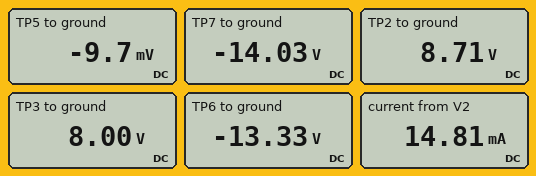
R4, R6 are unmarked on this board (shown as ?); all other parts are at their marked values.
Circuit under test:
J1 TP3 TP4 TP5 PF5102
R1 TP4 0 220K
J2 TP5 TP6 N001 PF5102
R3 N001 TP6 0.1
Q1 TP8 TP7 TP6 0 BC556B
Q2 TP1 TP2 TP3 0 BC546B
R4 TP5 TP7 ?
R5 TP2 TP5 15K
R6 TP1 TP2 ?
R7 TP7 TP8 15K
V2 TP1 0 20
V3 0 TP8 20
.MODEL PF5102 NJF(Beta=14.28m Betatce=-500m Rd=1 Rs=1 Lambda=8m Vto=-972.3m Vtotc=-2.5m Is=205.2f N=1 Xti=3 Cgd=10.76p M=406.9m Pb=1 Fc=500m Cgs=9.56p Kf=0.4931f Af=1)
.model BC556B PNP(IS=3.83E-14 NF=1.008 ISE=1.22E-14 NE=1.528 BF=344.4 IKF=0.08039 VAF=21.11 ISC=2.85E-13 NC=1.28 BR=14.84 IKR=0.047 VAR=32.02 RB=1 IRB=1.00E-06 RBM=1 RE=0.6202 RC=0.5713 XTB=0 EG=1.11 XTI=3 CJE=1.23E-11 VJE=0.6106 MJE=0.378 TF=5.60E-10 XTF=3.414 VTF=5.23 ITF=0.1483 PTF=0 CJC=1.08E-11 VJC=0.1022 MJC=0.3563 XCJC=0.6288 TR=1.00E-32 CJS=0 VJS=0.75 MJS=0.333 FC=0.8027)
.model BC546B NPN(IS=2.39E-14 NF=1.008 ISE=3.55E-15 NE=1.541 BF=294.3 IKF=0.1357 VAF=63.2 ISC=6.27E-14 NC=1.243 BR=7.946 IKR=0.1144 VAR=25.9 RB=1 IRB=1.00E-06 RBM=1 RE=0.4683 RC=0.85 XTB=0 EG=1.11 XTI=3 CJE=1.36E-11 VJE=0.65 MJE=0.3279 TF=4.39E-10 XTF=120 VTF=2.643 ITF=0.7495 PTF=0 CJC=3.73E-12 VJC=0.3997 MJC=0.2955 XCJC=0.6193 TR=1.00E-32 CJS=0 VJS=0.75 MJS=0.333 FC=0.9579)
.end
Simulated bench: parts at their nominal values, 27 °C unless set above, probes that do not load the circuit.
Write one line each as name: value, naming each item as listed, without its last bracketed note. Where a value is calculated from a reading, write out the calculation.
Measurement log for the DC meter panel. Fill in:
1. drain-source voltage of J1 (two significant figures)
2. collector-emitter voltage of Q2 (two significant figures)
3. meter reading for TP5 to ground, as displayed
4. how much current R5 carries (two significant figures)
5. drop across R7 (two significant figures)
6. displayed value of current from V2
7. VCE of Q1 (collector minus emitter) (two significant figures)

drain-source voltage of J1: 8 V - (-9.7 mV) = 8.0 V
collector-emitter voltage of Q2: 20 V - 8 V = 12 V
meter reading for TP5 to ground, as displayed: -9.7 mV
how much current R5 carries: (8.71 V - (-9.7 mV)) / 15 kΩ = 580 µA
drop across R7: -14.03 V - (-20 V) = 6.0 V
displayed value of current from V2: 14.81 mA
VCE of Q1 (collector minus emitter): -20 V - (-13.33 V) = -6.7 V
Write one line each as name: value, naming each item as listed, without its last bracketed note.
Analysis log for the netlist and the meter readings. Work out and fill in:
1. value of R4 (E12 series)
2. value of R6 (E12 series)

value of R4: 39 kΩ
value of R6: 18 kΩ
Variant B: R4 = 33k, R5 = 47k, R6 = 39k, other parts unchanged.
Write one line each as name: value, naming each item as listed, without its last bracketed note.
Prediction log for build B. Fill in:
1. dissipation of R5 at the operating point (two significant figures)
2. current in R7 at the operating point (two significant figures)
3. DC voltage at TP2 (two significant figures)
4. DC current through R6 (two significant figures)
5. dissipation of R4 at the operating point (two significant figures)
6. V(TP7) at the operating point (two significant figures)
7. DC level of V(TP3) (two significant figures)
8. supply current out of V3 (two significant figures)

dissipation of R5 at the operating point: 2.1 mW
current in R7 at the operating point: 440 µA
DC voltage at TP2: 9.9 V
DC current through R6: 260 µA
dissipation of R4 at the operating point: 5.4 mW
V(TP7) at the operating point: -13 V
DC level of V(TP3): 9.2 V
supply current out of V3: 15 mA
